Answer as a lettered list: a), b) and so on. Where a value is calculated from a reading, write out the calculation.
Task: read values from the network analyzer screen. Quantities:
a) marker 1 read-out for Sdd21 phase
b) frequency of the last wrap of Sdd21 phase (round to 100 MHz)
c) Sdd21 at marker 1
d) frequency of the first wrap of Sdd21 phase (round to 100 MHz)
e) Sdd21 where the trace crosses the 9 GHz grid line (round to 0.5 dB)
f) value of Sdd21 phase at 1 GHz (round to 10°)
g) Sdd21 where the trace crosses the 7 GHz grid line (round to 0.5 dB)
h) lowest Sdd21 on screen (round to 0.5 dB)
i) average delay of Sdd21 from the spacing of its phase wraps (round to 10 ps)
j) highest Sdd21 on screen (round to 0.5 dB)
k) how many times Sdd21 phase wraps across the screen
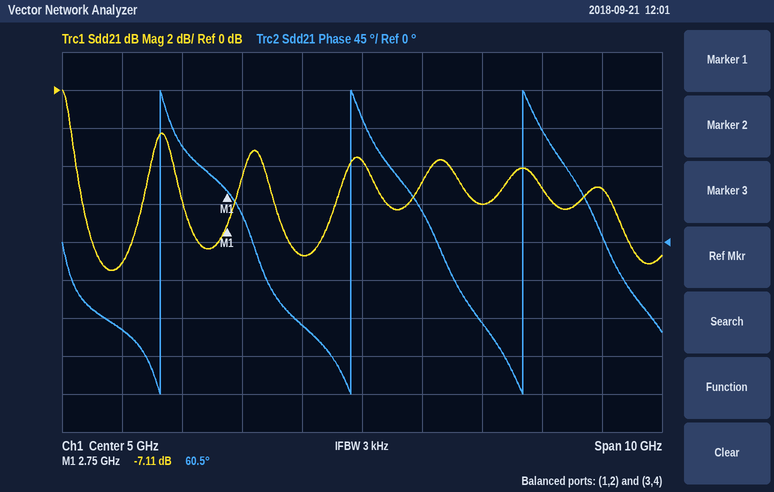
a) 60.5°
b) 7.7 GHz
c) -7.11 dB
d) 1.6 GHz
e) -5.0 dB
f) -100°
g) -6.0 dB
h) -9.5 dB
i) 2 cycles / (7.7 GHz − 1.6 GHz) ≈ 328 ps, so 330 ps to the nearest 10 ps
j) 0.0 dB
k) 3
